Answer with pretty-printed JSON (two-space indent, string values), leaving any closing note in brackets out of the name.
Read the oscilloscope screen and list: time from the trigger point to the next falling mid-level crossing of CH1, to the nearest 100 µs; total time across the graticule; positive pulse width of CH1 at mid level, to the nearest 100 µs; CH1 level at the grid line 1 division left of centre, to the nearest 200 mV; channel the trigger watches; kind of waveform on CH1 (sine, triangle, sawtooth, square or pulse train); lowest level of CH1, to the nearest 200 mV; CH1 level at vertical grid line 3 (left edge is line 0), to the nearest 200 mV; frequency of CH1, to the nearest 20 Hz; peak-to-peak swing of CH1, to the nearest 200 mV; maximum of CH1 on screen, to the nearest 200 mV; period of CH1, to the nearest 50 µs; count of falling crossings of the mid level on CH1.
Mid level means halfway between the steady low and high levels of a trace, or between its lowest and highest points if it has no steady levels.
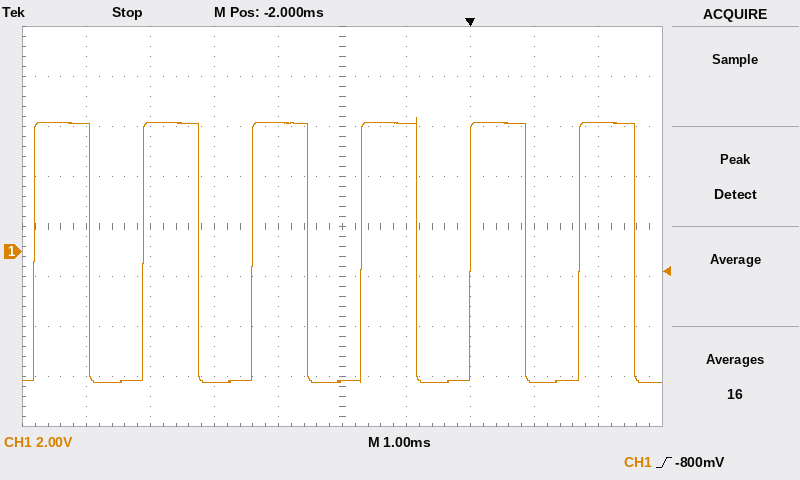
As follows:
{
  "time from the trigger point to the next falling mid-level crossing of CH1, to the nearest 100 µs": "900 µs",
  "total time across the graticule": "10 ms",
  "positive pulse width of CH1 at mid level, to the nearest 100 µs": "900 µs",
  "CH1 level at the grid line 1 division left of centre, to the nearest 200 mV": "5.2 V",
  "channel the trigger watches": "CH1",
  "kind of waveform on CH1": "square",
  "lowest level of CH1, to the nearest 200 mV": "-5.2 V",
  "CH1 level at vertical grid line 3 (left edge is line 0), to the nearest 200 mV": "-5.2 V",
  "frequency of CH1, to the nearest 20 Hz": "580 Hz",
  "peak-to-peak swing of CH1, to the nearest 200 mV": "10.6 V",
  "maximum of CH1 on screen, to the nearest 200 mV": "5.4 V",
  "period of CH1, to the nearest 50 µs": "1.70 ms",
  "count of falling crossings of the mid level on CH1": "6"
}
